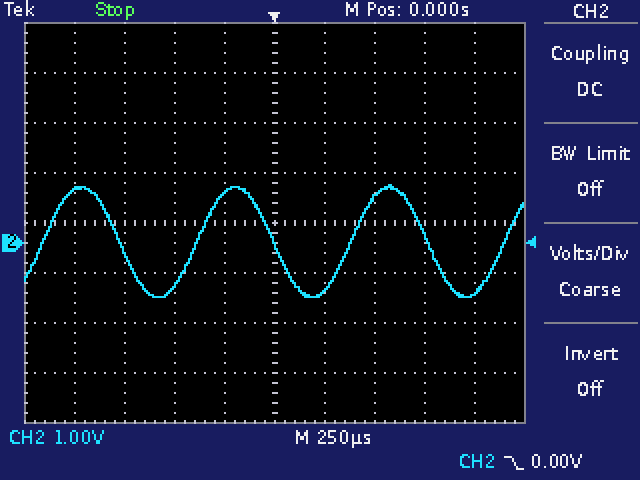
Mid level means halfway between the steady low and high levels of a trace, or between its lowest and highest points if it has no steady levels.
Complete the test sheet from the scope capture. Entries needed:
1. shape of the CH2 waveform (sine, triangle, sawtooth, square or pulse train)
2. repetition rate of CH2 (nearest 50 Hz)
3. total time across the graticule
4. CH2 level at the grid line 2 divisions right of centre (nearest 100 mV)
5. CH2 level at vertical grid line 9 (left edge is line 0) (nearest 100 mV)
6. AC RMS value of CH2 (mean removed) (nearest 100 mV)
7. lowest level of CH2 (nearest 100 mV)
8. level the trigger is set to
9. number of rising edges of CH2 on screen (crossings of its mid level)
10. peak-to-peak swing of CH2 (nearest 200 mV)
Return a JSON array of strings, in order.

["sine", "1.30 kHz", "2.5 ms", "900 mV", "-1.0 V", "800 mV", "-1.1 V", "0.00 V", "4", "2.2 V"]
